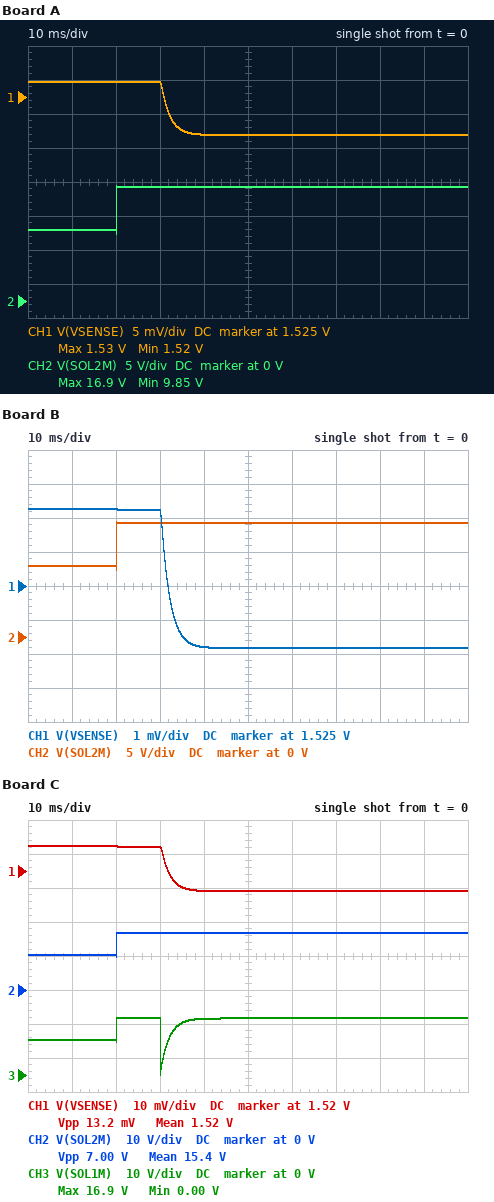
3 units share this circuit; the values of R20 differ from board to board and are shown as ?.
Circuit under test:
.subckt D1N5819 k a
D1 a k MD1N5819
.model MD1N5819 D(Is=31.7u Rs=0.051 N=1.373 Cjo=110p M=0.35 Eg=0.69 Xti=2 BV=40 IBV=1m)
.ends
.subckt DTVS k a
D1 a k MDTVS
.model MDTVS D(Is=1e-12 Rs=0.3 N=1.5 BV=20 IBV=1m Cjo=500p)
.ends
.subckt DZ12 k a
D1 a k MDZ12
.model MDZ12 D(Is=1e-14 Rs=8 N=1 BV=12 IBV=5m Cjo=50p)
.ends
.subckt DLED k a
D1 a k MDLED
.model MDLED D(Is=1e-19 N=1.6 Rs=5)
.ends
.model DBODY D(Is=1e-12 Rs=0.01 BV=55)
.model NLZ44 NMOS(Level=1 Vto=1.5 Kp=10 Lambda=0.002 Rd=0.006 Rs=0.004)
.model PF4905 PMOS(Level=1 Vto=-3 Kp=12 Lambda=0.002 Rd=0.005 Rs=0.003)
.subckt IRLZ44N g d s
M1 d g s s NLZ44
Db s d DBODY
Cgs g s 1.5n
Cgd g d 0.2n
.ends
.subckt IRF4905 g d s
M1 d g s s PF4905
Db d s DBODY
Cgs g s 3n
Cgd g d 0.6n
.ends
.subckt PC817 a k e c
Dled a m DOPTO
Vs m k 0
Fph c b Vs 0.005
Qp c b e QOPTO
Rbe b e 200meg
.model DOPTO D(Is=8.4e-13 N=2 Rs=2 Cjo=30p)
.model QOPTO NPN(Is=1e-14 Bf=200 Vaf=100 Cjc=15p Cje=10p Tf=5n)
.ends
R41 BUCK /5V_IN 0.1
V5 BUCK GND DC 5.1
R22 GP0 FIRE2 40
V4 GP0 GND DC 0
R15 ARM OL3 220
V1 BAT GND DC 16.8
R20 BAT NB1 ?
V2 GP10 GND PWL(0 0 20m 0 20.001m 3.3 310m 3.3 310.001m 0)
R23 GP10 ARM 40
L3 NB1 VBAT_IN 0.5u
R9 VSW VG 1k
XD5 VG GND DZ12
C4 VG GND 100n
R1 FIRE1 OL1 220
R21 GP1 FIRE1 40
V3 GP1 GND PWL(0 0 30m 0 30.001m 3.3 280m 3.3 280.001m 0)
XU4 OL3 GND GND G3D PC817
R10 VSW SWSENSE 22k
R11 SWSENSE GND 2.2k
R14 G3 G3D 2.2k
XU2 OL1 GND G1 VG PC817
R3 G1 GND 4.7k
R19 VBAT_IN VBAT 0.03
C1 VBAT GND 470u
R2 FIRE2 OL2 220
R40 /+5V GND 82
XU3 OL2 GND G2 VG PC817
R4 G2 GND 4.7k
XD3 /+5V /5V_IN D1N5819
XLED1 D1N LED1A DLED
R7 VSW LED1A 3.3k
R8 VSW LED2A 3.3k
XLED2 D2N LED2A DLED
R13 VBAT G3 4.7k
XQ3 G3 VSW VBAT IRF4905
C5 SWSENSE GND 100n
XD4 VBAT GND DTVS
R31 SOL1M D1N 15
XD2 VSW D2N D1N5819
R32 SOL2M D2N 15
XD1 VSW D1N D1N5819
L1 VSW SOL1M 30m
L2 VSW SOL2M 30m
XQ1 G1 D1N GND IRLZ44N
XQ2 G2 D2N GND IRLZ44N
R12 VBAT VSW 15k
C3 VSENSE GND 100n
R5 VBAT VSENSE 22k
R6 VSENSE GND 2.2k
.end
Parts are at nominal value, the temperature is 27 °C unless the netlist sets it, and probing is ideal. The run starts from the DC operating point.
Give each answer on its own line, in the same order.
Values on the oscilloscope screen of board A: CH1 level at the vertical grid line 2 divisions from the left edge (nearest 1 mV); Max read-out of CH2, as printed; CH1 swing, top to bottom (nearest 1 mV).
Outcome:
1.527 V
16.9 V
8 mV
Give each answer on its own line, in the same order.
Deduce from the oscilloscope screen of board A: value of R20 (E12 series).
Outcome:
0.047 Ω
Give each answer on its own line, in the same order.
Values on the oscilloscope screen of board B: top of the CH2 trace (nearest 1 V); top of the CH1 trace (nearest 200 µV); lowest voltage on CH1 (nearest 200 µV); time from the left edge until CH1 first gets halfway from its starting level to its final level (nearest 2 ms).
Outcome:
17 V
1.5272 V
1.5232 V
32 ms
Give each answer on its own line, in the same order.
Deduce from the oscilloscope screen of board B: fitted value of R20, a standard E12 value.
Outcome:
0.01 Ω
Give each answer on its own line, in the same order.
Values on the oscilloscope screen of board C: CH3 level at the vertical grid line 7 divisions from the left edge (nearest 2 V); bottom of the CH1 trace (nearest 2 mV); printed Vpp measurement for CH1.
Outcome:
16 V
1.514 V
13.2 mV
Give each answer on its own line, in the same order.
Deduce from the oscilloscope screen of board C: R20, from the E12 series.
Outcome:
0.1 Ω
